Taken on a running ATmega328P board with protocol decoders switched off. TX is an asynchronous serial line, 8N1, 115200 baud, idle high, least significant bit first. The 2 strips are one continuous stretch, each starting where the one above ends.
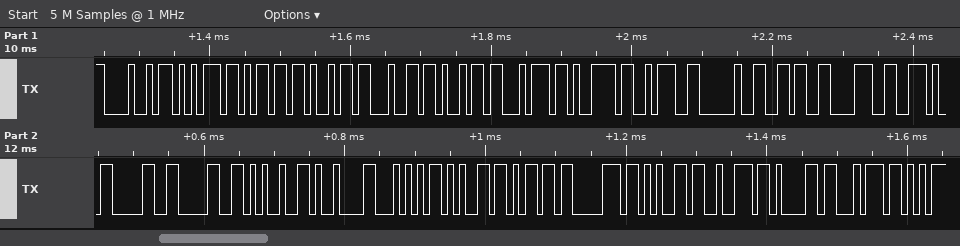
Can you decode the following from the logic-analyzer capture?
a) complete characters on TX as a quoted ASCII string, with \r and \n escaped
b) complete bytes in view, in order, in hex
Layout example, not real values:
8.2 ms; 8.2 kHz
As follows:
"Humidity: 68.00%\tTemperat"; 48 75 6D 69 64 69 74 79 3A 20 36 38 2E 30 30 25 09 54 65 6D 70 65 72 61 74
